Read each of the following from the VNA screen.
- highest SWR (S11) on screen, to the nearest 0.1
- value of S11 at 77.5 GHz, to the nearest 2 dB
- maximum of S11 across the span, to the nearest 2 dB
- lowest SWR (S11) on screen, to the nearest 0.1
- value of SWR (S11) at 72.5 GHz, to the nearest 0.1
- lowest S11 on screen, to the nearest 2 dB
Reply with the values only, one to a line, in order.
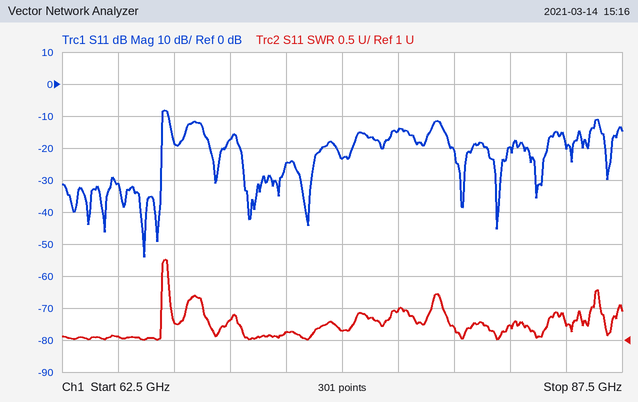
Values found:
2.3
-14 dB
-8 dB
1.0
1.1
-54 dB
